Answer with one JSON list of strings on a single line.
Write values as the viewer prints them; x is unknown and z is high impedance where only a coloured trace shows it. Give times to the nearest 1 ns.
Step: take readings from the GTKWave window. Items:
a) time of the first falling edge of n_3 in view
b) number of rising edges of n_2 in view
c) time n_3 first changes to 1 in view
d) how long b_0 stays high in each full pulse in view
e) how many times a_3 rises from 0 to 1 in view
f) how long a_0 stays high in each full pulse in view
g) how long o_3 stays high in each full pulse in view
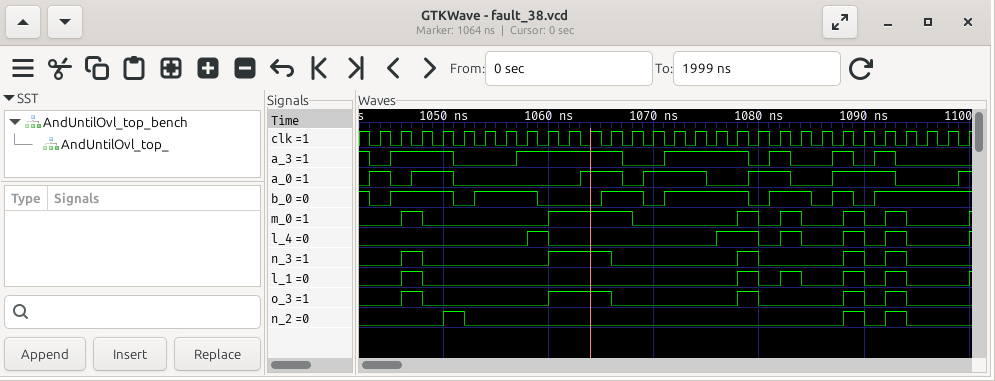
["1048 ns", "3", "1046 ns", "6 ns, 6 ns, 4 ns, 8 ns, 4 ns, 2 ns", "6", "2 ns, 4 ns, 4 ns, 6 ns, 4 ns, 6 ns", "2 ns, 6 ns, 2 ns, 2 ns, 2 ns"]
